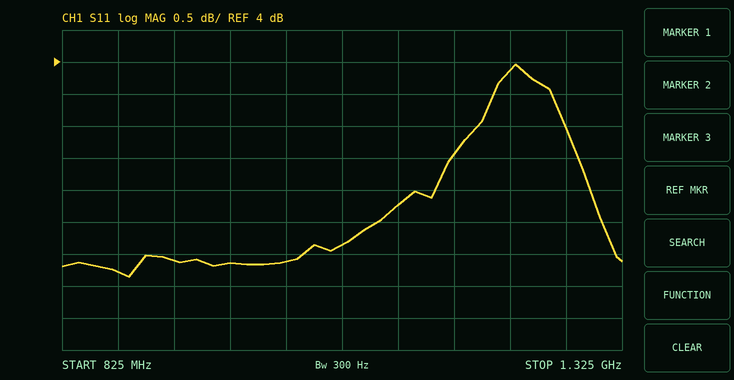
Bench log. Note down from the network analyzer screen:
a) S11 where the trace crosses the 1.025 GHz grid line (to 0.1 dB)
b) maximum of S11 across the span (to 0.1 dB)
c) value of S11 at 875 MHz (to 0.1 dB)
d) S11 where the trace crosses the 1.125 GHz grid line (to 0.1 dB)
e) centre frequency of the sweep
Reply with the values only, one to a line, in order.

0.9 dB
4.0 dB
0.7 dB
1.8 dB
1.075 GHz
